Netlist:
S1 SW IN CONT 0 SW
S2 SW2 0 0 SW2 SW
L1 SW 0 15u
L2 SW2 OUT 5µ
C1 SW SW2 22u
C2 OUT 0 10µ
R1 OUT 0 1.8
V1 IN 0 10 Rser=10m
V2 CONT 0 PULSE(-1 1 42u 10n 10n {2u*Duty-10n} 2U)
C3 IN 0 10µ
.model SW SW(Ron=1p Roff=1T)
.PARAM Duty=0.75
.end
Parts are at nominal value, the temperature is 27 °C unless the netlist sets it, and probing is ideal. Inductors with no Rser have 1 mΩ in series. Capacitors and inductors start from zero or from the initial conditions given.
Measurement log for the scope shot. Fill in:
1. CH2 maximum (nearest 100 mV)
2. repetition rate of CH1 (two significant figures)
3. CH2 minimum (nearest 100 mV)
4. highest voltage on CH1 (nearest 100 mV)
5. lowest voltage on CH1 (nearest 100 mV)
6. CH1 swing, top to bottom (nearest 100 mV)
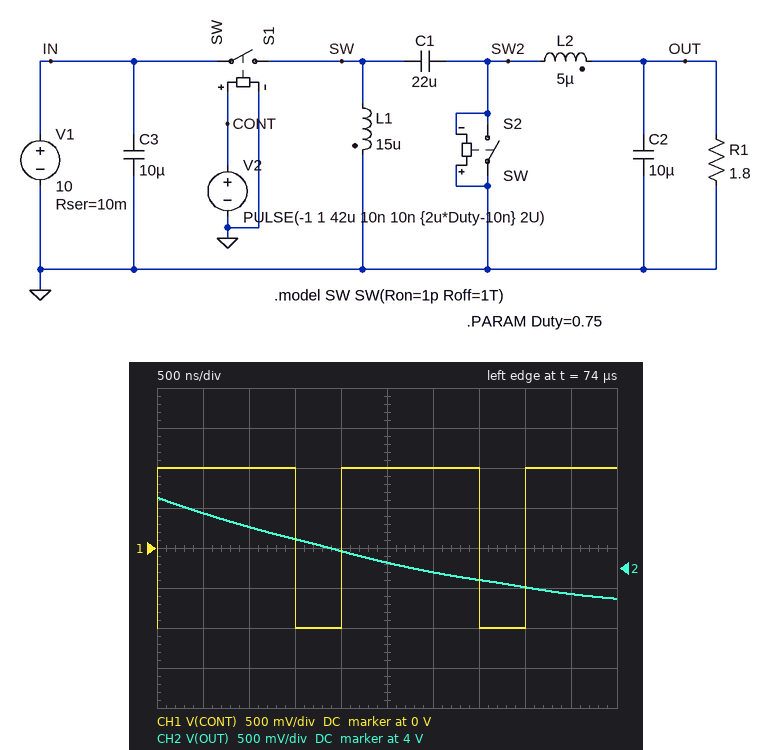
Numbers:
4.9 V
500 kHz
3.6 V
1.0 V
-1.0 V
2.0 V
